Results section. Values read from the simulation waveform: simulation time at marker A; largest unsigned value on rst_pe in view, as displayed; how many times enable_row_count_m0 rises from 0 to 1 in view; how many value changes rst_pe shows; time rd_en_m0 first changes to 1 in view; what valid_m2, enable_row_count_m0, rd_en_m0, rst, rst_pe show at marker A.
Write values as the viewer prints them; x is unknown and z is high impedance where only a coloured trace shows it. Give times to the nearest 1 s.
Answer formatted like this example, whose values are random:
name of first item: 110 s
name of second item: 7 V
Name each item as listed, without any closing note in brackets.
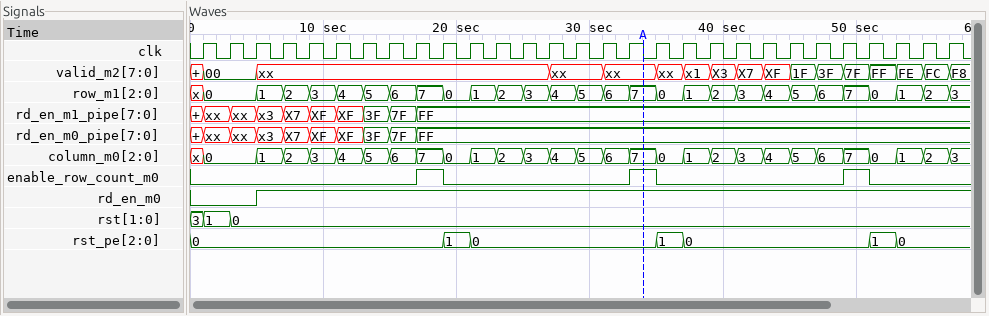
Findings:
simulation time at marker A: 34 s
largest unsigned value on rst_pe in view, as displayed: 1
how many times enable_row_count_m0 rises from 0 to 1 in view: 3
how many value changes rst_pe shows: 6
time rd_en_m0 first changes to 1 in view: 5 s
what valid_m2, enable_row_count_m0, rd_en_m0, rst, rst_pe show at marker A: valid_m2=xx, enable_row_count_m0=1, rd_en_m0=1, rst=0, rst_pe=0
